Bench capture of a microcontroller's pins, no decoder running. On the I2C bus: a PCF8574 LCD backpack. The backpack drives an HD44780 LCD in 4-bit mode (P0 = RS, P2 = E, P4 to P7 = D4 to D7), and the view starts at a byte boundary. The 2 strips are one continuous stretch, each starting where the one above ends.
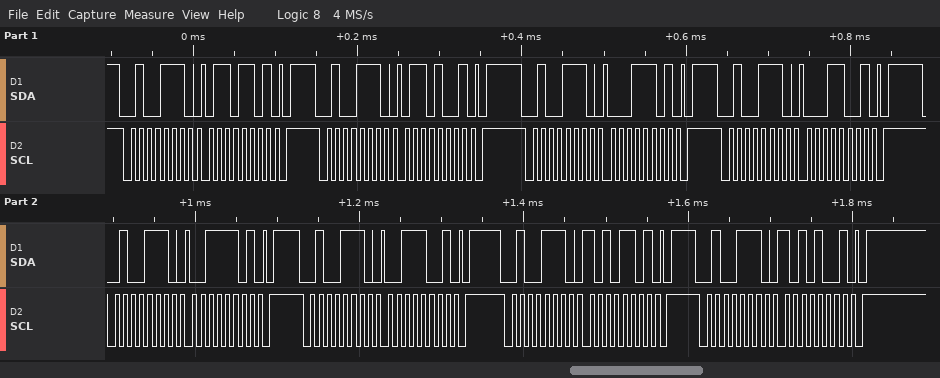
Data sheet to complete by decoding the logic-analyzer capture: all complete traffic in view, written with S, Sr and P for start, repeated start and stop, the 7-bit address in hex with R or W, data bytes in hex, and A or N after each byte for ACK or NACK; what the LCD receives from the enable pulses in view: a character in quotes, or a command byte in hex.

S 27W A 6D A P S 27W A 69 A P S 27W A 1D A P S 27W A 19 A P S 27W A 3D A P S 27W A 39 A P S 27W A AD A P S 27W A A9 A P
'a' ':'
